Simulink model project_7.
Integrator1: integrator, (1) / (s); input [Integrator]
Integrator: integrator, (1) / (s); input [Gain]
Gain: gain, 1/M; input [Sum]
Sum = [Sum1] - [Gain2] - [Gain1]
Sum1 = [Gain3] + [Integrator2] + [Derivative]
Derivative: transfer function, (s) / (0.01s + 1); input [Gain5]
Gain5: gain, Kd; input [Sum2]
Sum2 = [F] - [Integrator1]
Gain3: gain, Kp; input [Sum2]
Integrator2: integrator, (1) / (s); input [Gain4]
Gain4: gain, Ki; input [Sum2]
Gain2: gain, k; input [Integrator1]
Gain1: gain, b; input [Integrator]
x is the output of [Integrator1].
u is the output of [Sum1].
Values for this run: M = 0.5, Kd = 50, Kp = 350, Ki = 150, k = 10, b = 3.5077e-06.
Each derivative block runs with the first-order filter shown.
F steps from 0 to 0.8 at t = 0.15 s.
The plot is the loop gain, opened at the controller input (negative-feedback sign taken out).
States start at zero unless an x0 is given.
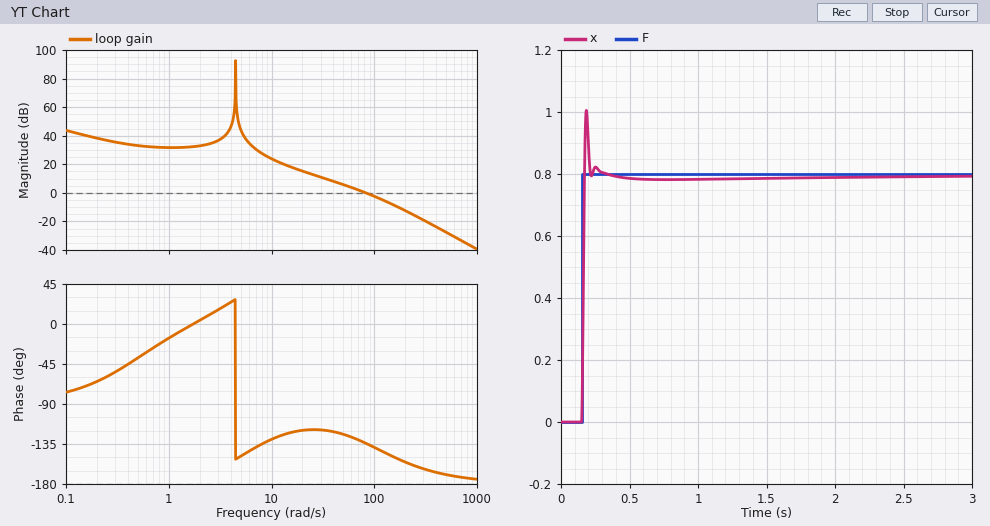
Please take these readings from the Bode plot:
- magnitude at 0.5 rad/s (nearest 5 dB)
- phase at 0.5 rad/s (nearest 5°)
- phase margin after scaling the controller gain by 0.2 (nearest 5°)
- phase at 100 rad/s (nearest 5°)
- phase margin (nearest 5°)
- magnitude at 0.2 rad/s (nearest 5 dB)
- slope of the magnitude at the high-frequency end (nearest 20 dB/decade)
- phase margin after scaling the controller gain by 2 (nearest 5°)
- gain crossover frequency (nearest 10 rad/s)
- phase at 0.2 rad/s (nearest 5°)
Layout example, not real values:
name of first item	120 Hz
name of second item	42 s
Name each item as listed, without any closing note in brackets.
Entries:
magnitude at 0.5 rad/s	35 dB
phase at 0.5 rad/s	-40°
phase margin after scaling the controller gain by 0.2	60°
phase at 100 rad/s	-140°
phase margin	45°
magnitude at 0.2 rad/s	40 dB
slope of the magnitude at the high-frequency end	-40 dB/decade
phase margin after scaling the controller gain by 2	35°
gain crossover frequency	80 rad/s
phase at 0.2 rad/s	-65°
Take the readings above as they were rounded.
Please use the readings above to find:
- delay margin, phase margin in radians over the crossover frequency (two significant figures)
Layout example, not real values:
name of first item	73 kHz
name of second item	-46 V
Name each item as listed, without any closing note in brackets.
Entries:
delay margin, phase margin in radians over the crossover frequency	0.0098 s
